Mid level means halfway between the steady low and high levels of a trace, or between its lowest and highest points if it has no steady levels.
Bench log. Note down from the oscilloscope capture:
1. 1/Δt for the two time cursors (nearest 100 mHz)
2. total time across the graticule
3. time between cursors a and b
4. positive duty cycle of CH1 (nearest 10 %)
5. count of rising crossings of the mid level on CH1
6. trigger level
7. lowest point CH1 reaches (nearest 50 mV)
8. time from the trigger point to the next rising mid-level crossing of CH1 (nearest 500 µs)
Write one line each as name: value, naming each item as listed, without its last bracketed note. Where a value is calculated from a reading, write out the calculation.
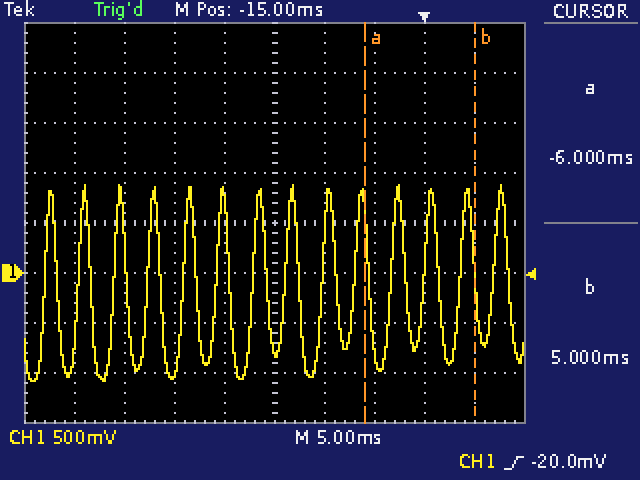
1/Δt for the two time cursors: 1 / 11.0 ms ≈ 90.9 Hz
total time across the graticule: 50 ms
time between cursors a and b: 5 ms − (-6 ms) = 11.0 ms
positive duty cycle of CH1: 40 %
count of rising crossings of the mid level on CH1: 14
trigger level: -20.0 mV
lowest point CH1 reaches: -1.10 V
time from the trigger point to the next rising mid-level crossing of CH1: 3.5 ms
